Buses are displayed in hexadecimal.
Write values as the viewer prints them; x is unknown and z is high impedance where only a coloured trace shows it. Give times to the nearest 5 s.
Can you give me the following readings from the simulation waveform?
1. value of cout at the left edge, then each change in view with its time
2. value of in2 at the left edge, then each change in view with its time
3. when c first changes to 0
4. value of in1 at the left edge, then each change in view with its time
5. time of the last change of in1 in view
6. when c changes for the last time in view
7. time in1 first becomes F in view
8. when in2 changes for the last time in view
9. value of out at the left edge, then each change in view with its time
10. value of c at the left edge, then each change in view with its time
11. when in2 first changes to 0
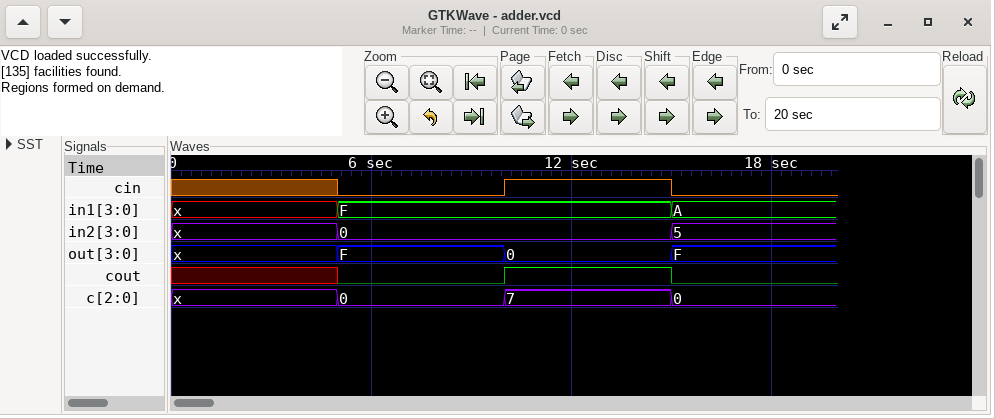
x, 0 at 5 s, 1 at 10 s, 0 at 15 s
x, 0 at 5 s, 5 at 15 s
5 s
x, F at 5 s, A at 15 s
15 s
15 s
5 s
15 s
x, F at 5 s, 0 at 10 s, F at 15 s
x, 0 at 5 s, 7 at 10 s, 0 at 15 s
5 s
